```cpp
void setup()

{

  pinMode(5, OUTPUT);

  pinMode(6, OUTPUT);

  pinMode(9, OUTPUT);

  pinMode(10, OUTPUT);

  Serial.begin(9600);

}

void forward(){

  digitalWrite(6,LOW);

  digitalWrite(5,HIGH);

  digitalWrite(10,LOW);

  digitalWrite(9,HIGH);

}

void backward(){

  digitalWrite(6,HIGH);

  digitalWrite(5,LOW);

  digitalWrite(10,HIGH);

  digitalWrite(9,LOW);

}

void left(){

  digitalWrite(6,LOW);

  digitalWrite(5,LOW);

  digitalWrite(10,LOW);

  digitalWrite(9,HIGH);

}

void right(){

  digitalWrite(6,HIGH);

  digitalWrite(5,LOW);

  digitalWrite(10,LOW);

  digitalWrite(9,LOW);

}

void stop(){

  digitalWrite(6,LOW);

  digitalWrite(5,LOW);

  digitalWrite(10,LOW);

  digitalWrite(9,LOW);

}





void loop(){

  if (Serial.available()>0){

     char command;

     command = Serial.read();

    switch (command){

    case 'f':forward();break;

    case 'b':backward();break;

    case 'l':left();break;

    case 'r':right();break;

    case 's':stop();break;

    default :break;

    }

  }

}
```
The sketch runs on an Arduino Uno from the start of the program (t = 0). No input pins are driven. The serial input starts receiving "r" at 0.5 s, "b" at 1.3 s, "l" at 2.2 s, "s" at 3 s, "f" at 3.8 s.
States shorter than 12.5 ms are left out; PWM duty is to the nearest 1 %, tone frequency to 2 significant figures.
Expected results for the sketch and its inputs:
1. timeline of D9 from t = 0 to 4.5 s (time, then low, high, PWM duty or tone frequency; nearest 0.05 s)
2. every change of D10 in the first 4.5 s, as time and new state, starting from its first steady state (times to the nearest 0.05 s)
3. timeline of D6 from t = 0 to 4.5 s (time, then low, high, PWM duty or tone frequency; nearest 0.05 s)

0 s low; 2.2 s high; 3 s low; 3.8 s high
0 s low; 1.3 s high; 2.2 s low
0 s low; 0.5 s high; 2.2 s low
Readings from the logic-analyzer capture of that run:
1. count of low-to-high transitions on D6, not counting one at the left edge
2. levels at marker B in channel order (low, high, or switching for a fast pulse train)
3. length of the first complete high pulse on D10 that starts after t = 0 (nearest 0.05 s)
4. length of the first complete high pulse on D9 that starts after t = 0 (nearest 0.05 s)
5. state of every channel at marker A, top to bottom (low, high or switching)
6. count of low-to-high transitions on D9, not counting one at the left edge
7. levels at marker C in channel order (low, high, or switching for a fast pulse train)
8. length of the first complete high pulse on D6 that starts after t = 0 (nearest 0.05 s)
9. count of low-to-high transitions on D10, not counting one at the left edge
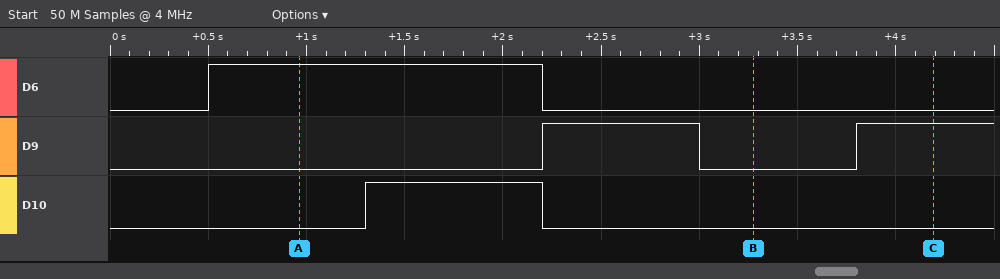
1
D6 low, D9 low, D10 low
0.90 s
0.80 s
D6 high, D9 low, D10 low
2
D6 low, D9 high, D10 low
1.70 s
1
